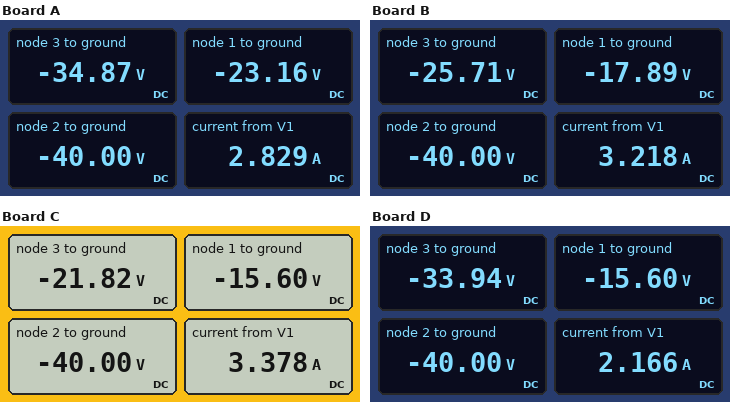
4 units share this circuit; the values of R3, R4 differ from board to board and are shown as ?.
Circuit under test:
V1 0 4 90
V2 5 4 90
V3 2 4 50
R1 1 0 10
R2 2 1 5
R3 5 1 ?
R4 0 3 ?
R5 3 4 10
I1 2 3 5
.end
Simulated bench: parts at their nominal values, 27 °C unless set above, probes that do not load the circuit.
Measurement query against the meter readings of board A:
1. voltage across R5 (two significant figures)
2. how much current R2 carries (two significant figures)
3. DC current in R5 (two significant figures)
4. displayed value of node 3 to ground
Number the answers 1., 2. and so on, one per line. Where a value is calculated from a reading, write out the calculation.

1. -34.87 V - (-90 V) = 55 V
2. (-23.16 V - (-40 V)) / 5 Ω = 3.4 A
3. (-34.87 V - (-90 V)) / 10 Ω = 5.5 A
4. -34.87 V
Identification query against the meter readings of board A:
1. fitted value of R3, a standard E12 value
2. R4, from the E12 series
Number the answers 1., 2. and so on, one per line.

1. 22 Ω
2. 68 Ω
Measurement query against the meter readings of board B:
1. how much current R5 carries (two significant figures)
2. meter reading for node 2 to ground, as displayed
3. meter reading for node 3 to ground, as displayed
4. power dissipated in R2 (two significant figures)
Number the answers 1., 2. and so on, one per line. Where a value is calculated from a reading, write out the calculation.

1. (-25.71 V - (-90 V)) / 10 Ω = 6.4 A
2. -40.00 V
3. -25.71 V
4. (-17.89 V - (-40 V))^2 / 5 Ω = 98 W
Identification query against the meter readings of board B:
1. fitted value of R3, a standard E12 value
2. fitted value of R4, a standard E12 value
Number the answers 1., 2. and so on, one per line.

1. 6.8 Ω
2. 18 Ω
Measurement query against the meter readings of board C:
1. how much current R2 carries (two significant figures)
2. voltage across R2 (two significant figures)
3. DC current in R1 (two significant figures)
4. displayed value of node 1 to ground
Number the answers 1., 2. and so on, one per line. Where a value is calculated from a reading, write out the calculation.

1. (-15.6 V - (-40 V)) / 5 Ω = 4.9 A
2. -15.6 V - (-40 V) = 24 V
3. (0 V - (-15.6 V)) / 10 Ω = 1.6 A
4. -15.60 V
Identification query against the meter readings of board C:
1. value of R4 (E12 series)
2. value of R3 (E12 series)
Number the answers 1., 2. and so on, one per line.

1. 12 Ω
2. 4.7 Ω
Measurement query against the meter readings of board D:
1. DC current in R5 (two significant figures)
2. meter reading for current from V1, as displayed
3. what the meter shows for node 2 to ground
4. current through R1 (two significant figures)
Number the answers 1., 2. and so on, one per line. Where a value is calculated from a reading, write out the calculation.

1. (-33.94 V - (-90 V)) / 10 Ω = 5.6 A
2. 2.166 A
3. -40.00 V
4. (0 V - (-15.6 V)) / 10 Ω = 1.6 A
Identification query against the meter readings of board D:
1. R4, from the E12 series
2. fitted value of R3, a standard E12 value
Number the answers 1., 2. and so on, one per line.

1. 56 Ω
2. 4.7 Ω
